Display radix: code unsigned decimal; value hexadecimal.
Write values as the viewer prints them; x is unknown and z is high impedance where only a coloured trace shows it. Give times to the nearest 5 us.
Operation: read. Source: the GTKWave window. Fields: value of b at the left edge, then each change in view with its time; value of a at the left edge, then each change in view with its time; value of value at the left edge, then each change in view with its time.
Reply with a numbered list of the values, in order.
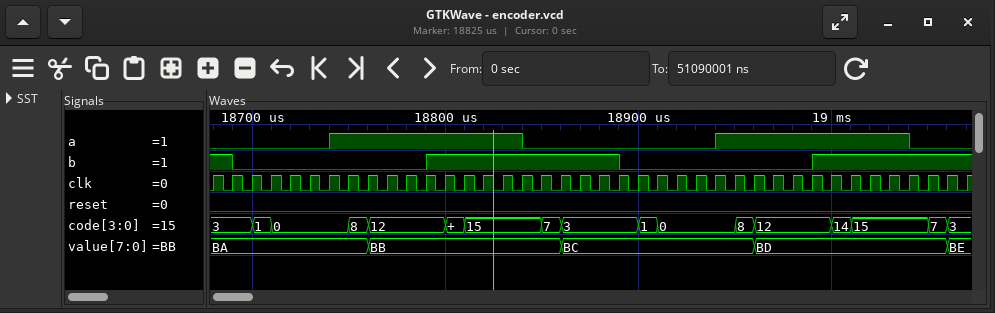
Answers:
1. 1, 0 at 18690 us, 1 at 18790 us, 0 at 18890 us, 1 at 18990 us
2. 0, 1 at 18740 us, 0 at 18840 us, 1 at 18940 us, 0 at 19040 us
3. BA, BB at 18760 us, BC at 18860 us, BD at 18960 us, BE at 19060 us
